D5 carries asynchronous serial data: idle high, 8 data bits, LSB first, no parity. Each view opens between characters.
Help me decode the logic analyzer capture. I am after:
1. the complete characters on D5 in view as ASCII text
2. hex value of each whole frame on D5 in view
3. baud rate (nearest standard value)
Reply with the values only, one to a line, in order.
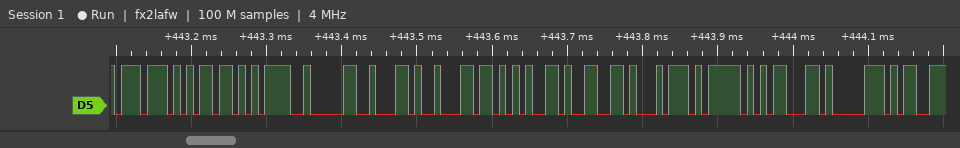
"wm=0,left_cp"
77, 6D, 3D, 30, 2C, 6C, 65, 66, 74, 5F, 63, 70
115200 baud
